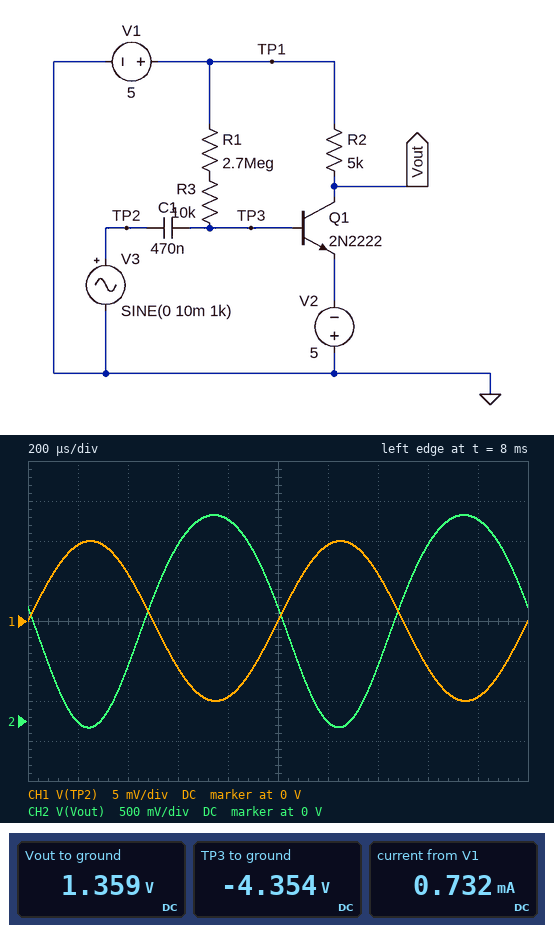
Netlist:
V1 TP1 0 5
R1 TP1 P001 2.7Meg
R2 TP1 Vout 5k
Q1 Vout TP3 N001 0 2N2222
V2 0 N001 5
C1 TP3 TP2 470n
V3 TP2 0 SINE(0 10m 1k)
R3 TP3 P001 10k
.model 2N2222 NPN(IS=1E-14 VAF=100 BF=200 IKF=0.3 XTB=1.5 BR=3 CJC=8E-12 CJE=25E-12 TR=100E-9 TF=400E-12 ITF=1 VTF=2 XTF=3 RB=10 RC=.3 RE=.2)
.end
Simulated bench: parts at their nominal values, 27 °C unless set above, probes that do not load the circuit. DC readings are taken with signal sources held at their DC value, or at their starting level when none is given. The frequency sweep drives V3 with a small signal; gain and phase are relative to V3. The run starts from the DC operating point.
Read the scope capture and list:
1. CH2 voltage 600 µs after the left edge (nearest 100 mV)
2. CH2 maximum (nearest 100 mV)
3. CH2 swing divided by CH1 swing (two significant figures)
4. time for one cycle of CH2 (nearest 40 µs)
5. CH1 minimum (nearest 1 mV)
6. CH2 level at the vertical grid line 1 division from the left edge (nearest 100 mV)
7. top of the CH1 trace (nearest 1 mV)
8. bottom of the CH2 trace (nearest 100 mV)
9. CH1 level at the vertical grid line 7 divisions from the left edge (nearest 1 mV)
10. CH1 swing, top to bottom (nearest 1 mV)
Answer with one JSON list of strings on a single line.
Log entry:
["2.2 V", "2.6 V", "130", "1.00 ms", "-10 mV", "0 V", "10 mV", "-100 mV", "6 mV", "20 mV"]
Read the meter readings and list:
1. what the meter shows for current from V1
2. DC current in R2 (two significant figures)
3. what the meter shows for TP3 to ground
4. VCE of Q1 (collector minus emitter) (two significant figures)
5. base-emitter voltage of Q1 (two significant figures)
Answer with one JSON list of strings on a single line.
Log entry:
["0.732 mA", "730 µA", "-4.354 V", "6.4 V", "650 mV"]
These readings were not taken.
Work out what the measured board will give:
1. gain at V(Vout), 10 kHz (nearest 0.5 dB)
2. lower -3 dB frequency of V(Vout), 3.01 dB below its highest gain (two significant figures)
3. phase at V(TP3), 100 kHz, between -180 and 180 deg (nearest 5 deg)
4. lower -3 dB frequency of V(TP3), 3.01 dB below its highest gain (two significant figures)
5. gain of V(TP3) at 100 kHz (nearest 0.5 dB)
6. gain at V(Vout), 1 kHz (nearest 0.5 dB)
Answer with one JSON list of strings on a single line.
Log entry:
["42.5 dB", "45 Hz", "0 deg", "45 Hz", "0 dB", "42.5 dB"]
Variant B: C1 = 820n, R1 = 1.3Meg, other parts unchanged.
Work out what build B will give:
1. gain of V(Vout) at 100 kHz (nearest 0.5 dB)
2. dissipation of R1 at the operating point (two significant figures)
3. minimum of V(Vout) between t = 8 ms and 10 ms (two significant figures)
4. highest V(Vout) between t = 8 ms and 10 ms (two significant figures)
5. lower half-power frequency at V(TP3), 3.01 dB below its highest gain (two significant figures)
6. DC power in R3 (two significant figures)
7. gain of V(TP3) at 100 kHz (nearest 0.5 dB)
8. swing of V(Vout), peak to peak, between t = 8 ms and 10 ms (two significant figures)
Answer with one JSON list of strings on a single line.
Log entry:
["48.0 dB", "66 µW", "-4.8 V", "140 mV", "53 Hz", "510 nW", "0 dB", "5.0 V"]
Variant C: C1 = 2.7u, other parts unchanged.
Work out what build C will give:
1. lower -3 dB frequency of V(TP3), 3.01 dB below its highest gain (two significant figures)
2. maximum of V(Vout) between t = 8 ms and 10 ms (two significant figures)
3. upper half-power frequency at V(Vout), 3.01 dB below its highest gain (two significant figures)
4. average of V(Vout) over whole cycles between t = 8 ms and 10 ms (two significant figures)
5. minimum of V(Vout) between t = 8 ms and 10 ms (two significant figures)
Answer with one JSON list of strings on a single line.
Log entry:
["7.8 Hz", "2.5 V", "6.5 MHz", "1.3 V", "-180 mV"]
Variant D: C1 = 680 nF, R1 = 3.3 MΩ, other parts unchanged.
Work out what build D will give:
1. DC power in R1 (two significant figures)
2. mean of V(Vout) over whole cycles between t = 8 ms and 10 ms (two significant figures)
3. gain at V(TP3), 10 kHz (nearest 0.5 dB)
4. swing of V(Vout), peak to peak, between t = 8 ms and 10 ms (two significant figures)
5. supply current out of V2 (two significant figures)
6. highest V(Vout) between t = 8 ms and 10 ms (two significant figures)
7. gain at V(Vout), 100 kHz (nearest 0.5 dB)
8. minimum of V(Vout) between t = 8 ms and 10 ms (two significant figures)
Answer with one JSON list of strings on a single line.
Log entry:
["26 µW", "2.0 V", "0 dB", "2.2 V", "600 µA", "3.0 V", "41.0 dB", "770 mV"]
